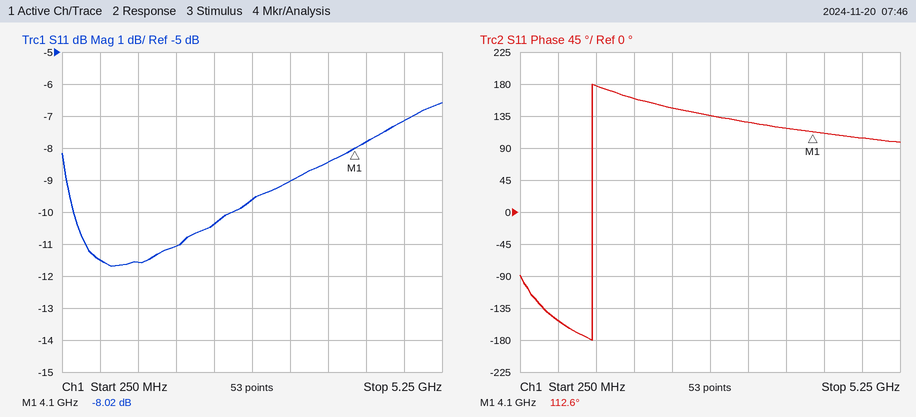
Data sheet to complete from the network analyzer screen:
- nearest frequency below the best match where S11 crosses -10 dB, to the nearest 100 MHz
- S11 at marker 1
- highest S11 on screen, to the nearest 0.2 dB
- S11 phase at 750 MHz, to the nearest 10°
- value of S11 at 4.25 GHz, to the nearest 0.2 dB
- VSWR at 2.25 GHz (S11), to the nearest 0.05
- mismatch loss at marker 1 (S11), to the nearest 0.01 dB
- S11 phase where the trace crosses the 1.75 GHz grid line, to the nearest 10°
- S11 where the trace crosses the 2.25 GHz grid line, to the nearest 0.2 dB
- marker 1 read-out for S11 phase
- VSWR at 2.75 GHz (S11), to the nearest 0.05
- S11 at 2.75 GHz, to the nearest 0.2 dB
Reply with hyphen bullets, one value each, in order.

- 400 MHz
- -8.02 dB
- -6.6 dB
- -150°
- -7.8 dB
- 1.85
- 0.75 dB
- 160°
- -10.4 dB
- 112.6°
- 2.00
- -9.6 dB
